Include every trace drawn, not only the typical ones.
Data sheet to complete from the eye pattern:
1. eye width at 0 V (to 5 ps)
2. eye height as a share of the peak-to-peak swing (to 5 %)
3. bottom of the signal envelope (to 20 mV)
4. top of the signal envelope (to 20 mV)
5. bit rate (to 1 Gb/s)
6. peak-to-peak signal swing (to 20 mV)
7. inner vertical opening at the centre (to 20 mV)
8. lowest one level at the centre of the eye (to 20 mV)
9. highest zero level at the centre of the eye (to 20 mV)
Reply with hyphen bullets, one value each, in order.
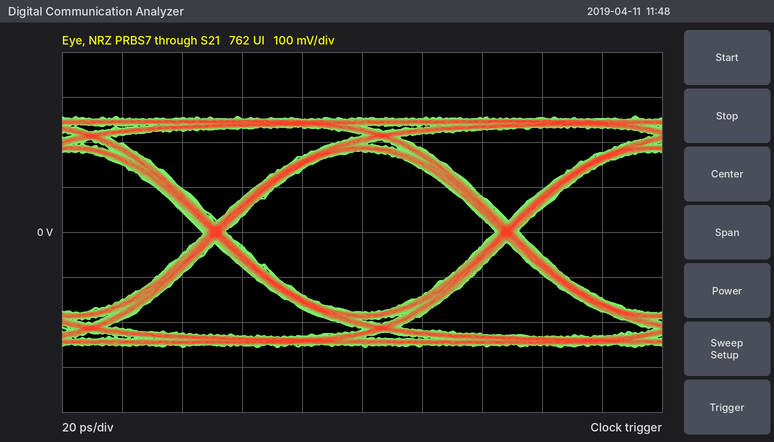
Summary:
- 90 ps
- 70 %
- -260 mV
- 260 mV
- 10 Gb/s
- 520 mV
- 360 mV
- 180 mV
- -180 mV
